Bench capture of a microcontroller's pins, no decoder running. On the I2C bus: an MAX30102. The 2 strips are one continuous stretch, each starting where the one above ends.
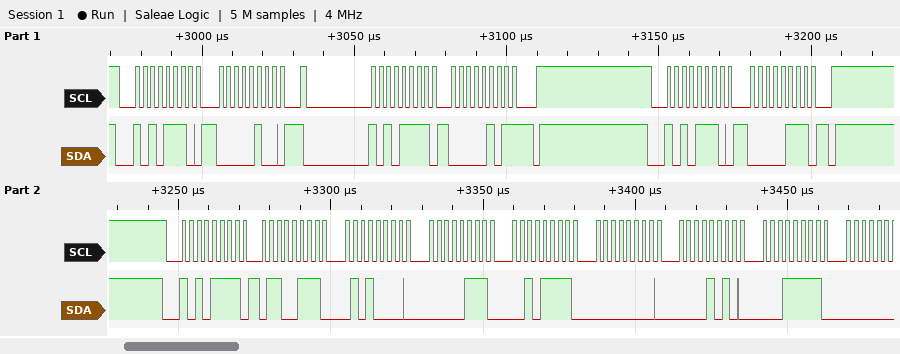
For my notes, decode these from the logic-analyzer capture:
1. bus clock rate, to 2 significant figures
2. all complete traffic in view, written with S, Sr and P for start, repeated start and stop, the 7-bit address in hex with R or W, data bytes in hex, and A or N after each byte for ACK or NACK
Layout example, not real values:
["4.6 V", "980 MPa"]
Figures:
["400 kHz", "S 57W A 04 A Sr 57R A 05 N P S 57W A 07 A P S 57R A 67 A 50 A 07 A 2F A 00 A 0A A 1F A"]
